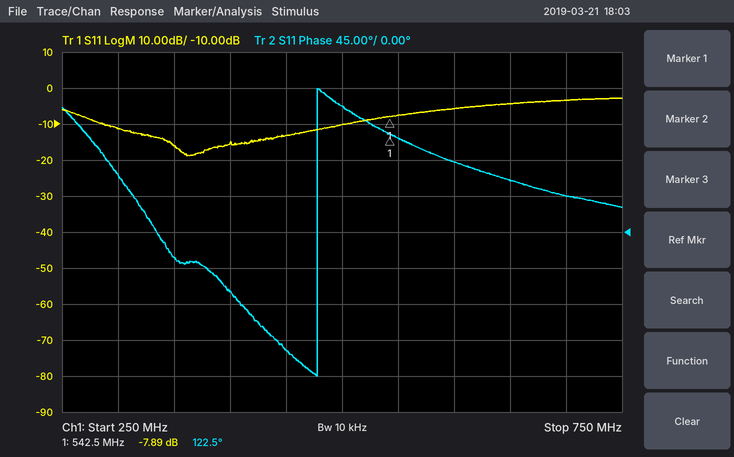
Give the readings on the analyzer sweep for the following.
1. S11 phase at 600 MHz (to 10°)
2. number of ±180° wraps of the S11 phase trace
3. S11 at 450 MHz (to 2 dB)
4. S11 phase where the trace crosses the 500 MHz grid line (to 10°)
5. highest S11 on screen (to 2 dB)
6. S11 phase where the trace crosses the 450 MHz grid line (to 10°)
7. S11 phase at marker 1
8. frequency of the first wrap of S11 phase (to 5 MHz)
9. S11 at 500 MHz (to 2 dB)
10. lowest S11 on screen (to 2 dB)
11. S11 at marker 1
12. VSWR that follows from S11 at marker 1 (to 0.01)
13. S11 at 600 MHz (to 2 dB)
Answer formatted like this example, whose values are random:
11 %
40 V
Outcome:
90°
1
-14 dB
160°
-2 dB
-150°
122.5°
480 MHz
-10 dB
-18 dB
-7.89 dB
2.35
-6 dB
